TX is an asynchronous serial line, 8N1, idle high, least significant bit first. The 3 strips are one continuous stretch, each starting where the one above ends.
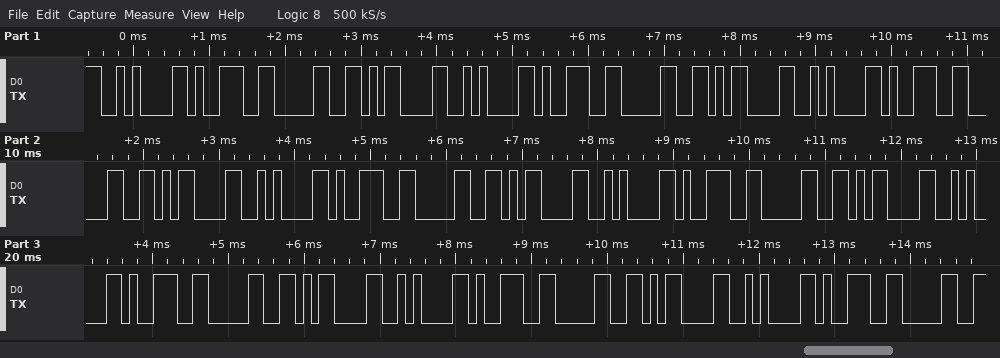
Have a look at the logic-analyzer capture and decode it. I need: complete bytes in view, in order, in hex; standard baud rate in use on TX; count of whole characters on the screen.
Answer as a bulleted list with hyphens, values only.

- 0A 39 30 0D 0A 39 30 0D 0A 39 30 0D 0A 39 30 0D 0A 39 30 0D 0A 39 30 0D 0A 39 30 0D 0A 39 30
- 9600 baud
- 31
